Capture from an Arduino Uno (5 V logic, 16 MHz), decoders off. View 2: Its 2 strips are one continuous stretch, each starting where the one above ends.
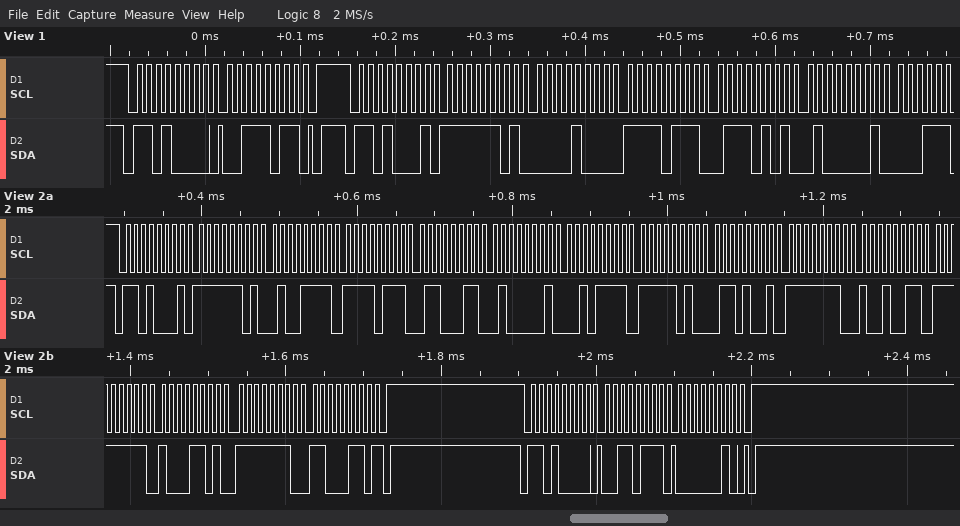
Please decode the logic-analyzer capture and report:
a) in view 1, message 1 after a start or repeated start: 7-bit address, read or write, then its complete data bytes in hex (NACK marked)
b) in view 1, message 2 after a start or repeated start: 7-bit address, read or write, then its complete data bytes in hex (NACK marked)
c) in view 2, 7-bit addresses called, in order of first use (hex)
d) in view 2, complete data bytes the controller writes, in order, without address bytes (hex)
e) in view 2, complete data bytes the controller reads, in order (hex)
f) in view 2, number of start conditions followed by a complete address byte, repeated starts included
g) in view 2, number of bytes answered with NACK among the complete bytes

0x68 write: 3B
0x68 read: FD 08 F7 75 41
0x68
37 02
FD 4F F7 63 41 2F FA 69 FE 93 FF 8D FE C6
2
1
